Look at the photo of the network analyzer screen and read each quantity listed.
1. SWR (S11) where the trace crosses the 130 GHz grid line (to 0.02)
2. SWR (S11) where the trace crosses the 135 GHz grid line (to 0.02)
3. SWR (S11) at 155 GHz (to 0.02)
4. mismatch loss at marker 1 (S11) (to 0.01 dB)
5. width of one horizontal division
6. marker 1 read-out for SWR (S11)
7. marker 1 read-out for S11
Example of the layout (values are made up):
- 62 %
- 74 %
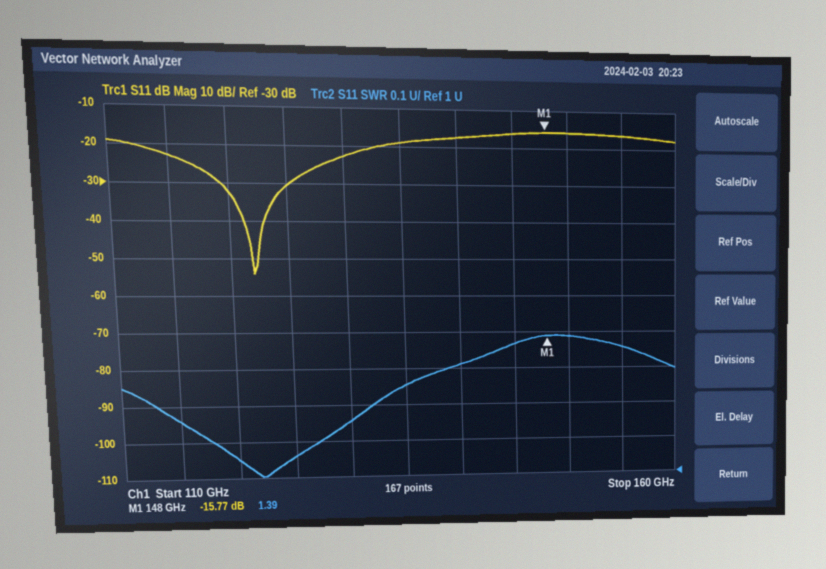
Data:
- 1.16
- 1.26
- 1.36
- 0.12 dB
- 5 GHz
- 1.39
- -15.77 dB
